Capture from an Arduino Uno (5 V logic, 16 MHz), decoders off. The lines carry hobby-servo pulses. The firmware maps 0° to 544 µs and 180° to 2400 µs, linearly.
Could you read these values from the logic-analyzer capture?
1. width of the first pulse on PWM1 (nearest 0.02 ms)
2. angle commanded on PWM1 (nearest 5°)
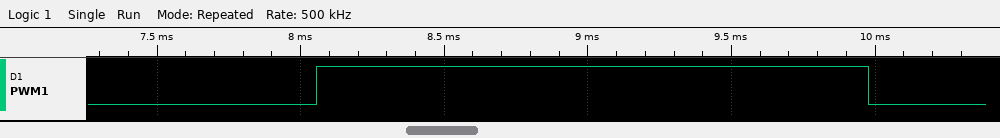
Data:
1.92 ms
135°
